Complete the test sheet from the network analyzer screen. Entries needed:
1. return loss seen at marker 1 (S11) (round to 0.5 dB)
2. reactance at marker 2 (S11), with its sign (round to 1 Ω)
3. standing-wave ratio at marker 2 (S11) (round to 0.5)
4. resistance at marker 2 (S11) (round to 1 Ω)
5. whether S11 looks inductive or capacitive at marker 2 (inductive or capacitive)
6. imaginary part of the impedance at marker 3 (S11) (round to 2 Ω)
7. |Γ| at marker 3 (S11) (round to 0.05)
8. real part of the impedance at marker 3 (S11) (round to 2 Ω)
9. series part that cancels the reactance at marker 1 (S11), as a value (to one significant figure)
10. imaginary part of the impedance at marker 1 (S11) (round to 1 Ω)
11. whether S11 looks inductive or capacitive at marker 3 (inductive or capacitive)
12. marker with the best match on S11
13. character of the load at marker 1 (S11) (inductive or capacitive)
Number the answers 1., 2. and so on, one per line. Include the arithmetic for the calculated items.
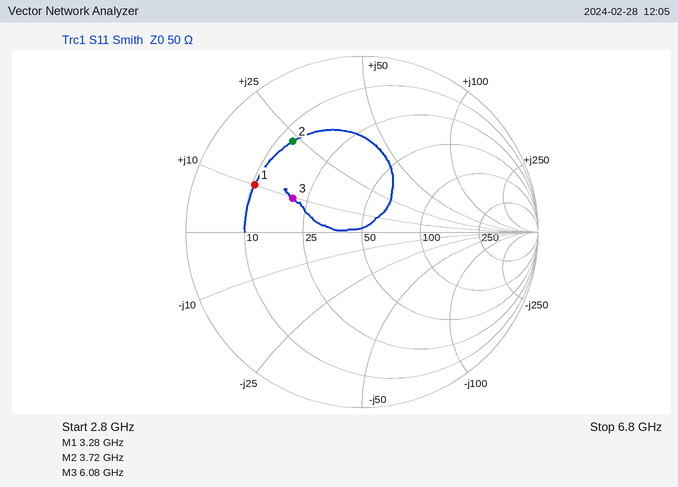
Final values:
1. 3.5 dB
2. +23 Ω
3. 4.5
4. 13 Ω
5. inductive
6. +10 Ω
7. 0.45
8. 20 Ω
9. C = 1/(2π × 3.28 GHz × 10 Ω) ≈ 5 pF
10. +10 Ω
11. inductive
12. marker 3
13. inductive
